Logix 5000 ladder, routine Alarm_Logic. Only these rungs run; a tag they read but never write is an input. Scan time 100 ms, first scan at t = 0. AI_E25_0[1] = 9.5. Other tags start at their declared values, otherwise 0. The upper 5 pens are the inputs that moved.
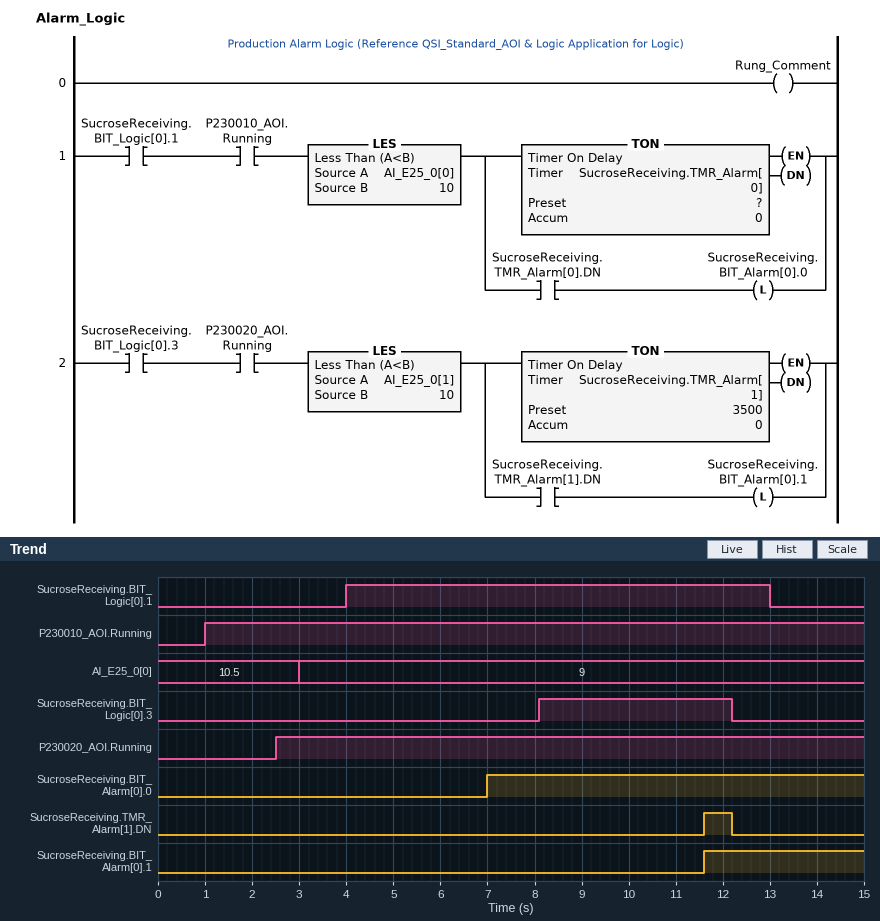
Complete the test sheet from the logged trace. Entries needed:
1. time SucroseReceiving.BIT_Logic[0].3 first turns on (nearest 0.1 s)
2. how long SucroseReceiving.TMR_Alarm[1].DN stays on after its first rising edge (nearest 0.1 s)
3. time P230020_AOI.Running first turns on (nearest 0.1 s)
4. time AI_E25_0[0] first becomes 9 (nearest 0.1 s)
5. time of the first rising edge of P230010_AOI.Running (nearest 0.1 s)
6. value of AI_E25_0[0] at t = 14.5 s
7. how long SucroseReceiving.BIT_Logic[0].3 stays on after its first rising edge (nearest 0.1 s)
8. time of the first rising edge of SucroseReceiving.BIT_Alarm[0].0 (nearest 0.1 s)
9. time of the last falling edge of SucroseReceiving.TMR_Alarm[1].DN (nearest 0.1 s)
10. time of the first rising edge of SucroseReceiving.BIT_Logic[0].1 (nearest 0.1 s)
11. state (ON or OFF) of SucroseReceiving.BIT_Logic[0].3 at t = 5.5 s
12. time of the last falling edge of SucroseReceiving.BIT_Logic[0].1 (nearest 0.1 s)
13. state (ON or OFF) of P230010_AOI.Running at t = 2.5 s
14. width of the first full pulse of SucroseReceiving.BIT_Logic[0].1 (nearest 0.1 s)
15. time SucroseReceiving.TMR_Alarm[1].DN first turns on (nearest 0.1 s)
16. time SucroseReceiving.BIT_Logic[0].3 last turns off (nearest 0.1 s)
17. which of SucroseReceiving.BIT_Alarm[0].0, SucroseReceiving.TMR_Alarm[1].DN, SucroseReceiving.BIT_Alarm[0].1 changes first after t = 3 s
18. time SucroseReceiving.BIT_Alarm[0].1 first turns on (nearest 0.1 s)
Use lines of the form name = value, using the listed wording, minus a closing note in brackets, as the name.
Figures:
time SucroseReceiving.BIT_Logic[0].3 first turns on = 8.1 s
how long SucroseReceiving.TMR_Alarm[1].DN stays on after its first rising edge = 0.6 s
time P230020_AOI.Running first turns on = 2.5 s
time AI_E25_0[0] first becomes 9 = 3.0 s
time of the first rising edge of P230010_AOI.Running = 1.0 s
value of AI_E25_0[0] at t = 14.5 s = 9
how long SucroseReceiving.BIT_Logic[0].3 stays on after its first rising edge = 4.1 s
time of the first rising edge of SucroseReceiving.BIT_Alarm[0].0 = 7.0 s
time of the last falling edge of SucroseReceiving.TMR_Alarm[1].DN = 12.2 s
time of the first rising edge of SucroseReceiving.BIT_Logic[0].1 = 4.0 s
state (ON or OFF) of SucroseReceiving.BIT_Logic[0].3 at t = 5.5 s = OFF
time of the last falling edge of SucroseReceiving.BIT_Logic[0].1 = 13.0 s
state (ON or OFF) of P230010_AOI.Running at t = 2.5 s = ON
width of the first full pulse of SucroseReceiving.BIT_Logic[0].1 = 9.0 s
time SucroseReceiving.TMR_Alarm[1].DN first turns on = 11.6 s
time SucroseReceiving.BIT_Logic[0].3 last turns off = 12.2 s
which of SucroseReceiving.BIT_Alarm[0].0, SucroseReceiving.TMR_Alarm[1].DN, SucroseReceiving.BIT_Alarm[0].1 changes first after t = 3 s = SucroseReceiving.BIT_Alarm[0].0
time SucroseReceiving.BIT_Alarm[0].1 first turns on = 11.6 s
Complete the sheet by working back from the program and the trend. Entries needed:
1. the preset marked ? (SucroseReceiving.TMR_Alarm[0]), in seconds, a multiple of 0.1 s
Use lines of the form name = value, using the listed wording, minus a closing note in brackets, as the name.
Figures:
the preset marked ? (SucroseReceiving.TMR_Alarm[0]), in seconds, a multiple of 0.1 s = 3.0 s
